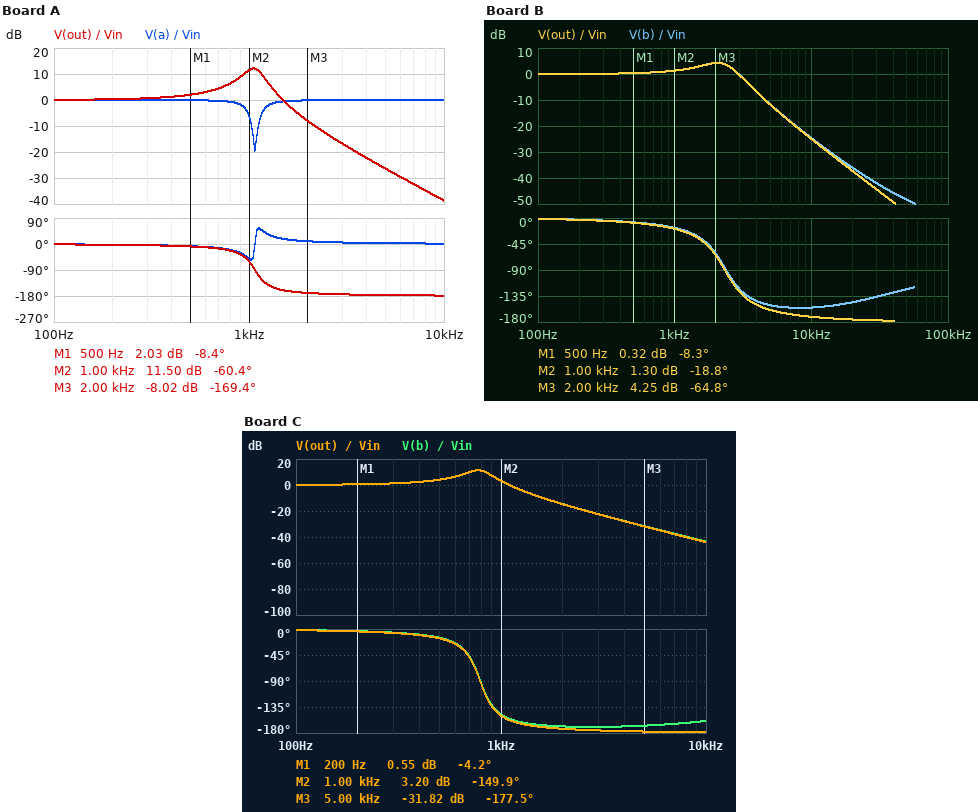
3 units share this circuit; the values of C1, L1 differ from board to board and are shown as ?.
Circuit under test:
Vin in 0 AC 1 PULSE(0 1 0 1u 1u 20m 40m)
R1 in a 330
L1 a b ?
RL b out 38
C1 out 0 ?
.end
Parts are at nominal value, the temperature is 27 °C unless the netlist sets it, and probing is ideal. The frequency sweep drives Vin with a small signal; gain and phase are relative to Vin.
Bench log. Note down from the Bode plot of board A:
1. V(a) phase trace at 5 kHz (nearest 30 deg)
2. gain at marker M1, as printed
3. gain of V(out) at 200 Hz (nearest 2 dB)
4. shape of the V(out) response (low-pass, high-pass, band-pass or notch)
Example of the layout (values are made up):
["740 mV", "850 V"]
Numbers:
["0 deg", "2.03 dB", "0 dB", "low-pass"]
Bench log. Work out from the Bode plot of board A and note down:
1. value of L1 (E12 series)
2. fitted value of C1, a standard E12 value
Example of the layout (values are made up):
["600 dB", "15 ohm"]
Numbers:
["220 mH", "100 nF"]
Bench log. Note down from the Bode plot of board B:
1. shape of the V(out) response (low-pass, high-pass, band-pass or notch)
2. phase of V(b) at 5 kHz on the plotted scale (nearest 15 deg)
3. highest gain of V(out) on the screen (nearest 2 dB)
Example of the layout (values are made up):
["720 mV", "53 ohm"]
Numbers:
["low-pass", "-150 deg", "4 dB"]
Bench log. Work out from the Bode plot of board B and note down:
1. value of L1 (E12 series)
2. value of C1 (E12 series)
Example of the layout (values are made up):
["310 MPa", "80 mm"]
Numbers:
["39 mH", "120 nF"]
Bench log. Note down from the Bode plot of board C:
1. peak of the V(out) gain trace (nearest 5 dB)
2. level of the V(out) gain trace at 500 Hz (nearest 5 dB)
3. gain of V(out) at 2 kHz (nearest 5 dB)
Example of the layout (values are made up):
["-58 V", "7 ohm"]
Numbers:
["10 dB", "5 dB", "-15 dB"]
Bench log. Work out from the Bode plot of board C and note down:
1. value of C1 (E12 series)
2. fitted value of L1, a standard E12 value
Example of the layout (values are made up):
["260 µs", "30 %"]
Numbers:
["150 nF", "270 mH"]
